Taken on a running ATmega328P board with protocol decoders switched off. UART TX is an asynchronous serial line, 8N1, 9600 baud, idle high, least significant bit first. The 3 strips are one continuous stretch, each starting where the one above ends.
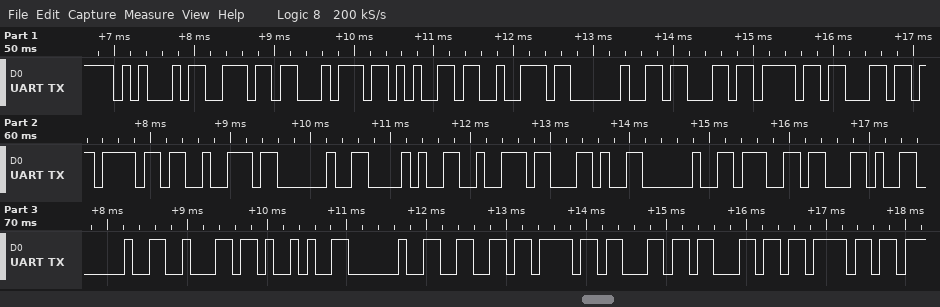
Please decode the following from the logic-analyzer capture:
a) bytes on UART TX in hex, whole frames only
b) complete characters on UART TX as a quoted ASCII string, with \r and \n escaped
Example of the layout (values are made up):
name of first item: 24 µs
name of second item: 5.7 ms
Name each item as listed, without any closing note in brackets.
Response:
bytes on UART TX in hex, whole frames only: 45 6E 74 65 72 20 63 6F 6C 6F 72 20 28 72 2C 20 67 2C 20 62 29 20 66 6F 6C 6C 6F
complete characters on UART TX as a quoted ASCII string, with \r and \n escaped: "Enter color (r, g, b) follo"
